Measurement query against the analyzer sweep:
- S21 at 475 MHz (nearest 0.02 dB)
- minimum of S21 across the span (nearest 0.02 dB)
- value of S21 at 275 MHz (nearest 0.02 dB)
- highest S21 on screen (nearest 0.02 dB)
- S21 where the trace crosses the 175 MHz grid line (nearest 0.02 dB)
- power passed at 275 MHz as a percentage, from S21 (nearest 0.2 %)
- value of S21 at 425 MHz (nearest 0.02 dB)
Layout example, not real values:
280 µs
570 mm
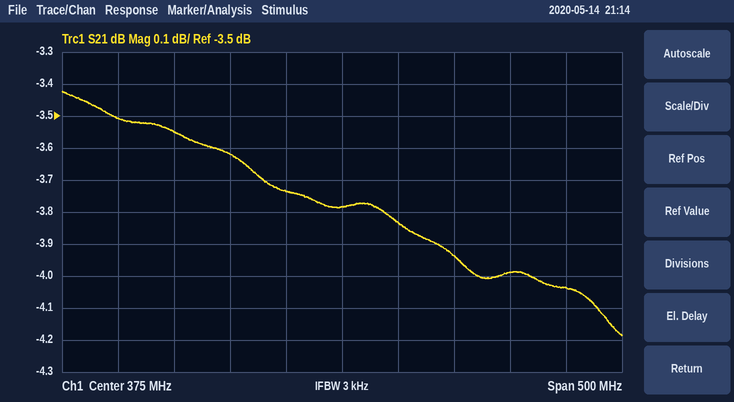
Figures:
-3.94 dB
-4.18 dB
-3.62 dB
-3.42 dB
-3.50 dB
43.4 %
-3.84 dB
